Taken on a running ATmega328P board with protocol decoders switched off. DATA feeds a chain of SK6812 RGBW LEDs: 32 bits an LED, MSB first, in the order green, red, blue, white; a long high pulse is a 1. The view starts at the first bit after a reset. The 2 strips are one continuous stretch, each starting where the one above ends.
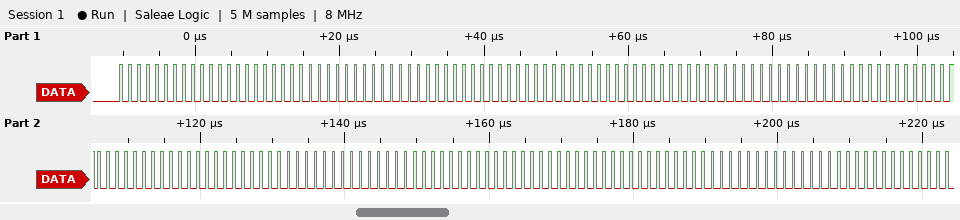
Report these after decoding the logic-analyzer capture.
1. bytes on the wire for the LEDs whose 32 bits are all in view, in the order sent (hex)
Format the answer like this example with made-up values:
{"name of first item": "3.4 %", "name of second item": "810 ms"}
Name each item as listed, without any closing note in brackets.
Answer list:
{"bytes on the wire for the LEDs whose 32 bits are all in view, in the order sent": "00 00 00 00 00 00 00 00 00 00 00 08 00 00 00 00 00 00 00 00"}
